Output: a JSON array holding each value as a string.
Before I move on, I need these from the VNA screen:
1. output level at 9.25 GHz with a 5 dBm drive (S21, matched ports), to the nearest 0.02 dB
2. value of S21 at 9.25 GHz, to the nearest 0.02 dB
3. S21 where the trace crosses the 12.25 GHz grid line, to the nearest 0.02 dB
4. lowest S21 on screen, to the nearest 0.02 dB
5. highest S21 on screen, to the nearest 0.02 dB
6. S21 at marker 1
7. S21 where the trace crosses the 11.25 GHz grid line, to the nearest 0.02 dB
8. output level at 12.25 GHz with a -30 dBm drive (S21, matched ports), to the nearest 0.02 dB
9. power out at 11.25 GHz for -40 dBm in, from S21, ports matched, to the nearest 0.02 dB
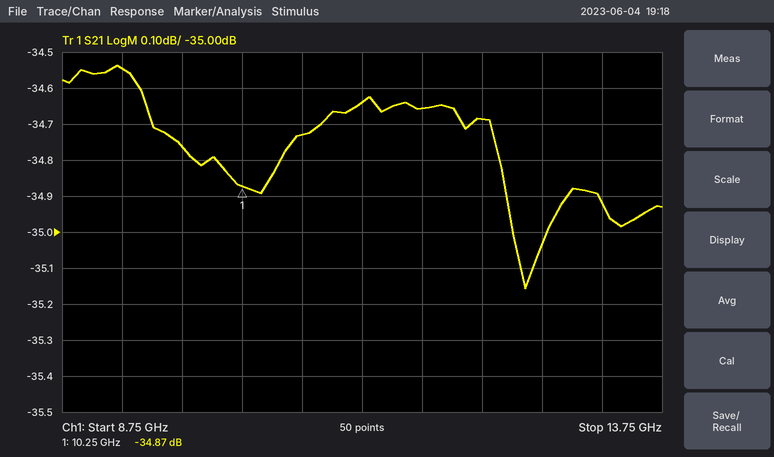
["-29.54 dBm", "-34.54 dB", "-34.68 dB", "-35.16 dB", "-34.54 dB", "-34.87 dB", "-34.64 dB", "-64.68 dBm", "-74.64 dBm"]
